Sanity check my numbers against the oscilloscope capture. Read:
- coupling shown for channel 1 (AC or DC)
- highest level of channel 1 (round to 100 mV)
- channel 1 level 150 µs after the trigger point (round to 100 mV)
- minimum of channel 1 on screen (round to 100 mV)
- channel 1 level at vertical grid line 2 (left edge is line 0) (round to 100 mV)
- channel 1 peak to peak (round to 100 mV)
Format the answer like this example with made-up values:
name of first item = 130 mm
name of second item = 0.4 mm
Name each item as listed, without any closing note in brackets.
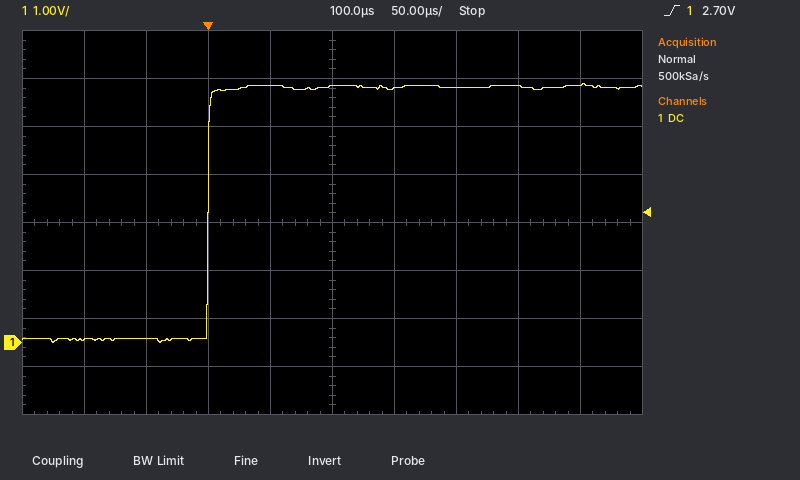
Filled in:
coupling shown for channel 1 = DC
highest level of channel 1 = 5.4 V
channel 1 level 150 µs after the trigger point = 5.3 V
minimum of channel 1 on screen = 0.0 V
channel 1 level at vertical grid line 2 (left edge is line 0) = 100 mV
channel 1 peak to peak = 5.4 V
